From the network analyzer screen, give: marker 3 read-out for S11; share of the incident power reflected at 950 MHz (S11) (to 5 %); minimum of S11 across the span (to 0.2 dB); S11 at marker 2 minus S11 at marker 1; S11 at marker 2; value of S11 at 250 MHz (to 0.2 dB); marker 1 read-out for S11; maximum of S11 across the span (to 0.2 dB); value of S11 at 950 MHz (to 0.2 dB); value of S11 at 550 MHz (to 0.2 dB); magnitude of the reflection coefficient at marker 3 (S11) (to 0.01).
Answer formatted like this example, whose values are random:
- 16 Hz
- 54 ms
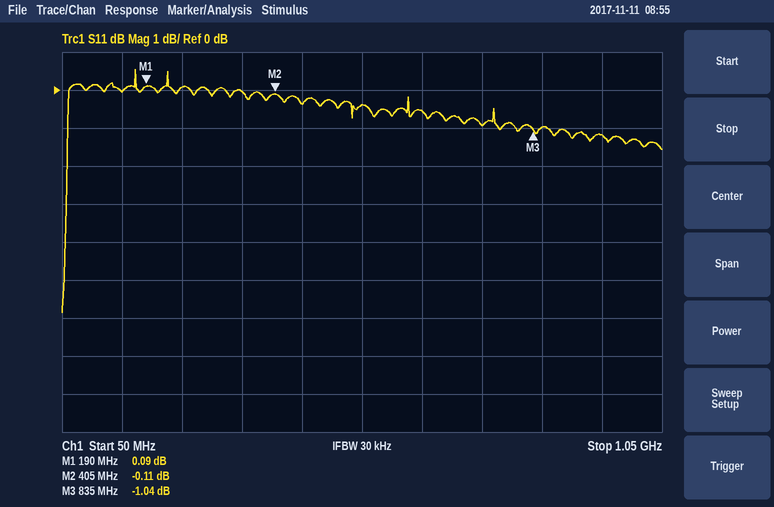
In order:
- -1.04 dB
- 75 %
- -5.8 dB
- -0.20 dB
- -0.11 dB
- 0.0 dB
- 0.09 dB
- 0.6 dB
- -1.2 dB
- -0.4 dB
- 0.89
